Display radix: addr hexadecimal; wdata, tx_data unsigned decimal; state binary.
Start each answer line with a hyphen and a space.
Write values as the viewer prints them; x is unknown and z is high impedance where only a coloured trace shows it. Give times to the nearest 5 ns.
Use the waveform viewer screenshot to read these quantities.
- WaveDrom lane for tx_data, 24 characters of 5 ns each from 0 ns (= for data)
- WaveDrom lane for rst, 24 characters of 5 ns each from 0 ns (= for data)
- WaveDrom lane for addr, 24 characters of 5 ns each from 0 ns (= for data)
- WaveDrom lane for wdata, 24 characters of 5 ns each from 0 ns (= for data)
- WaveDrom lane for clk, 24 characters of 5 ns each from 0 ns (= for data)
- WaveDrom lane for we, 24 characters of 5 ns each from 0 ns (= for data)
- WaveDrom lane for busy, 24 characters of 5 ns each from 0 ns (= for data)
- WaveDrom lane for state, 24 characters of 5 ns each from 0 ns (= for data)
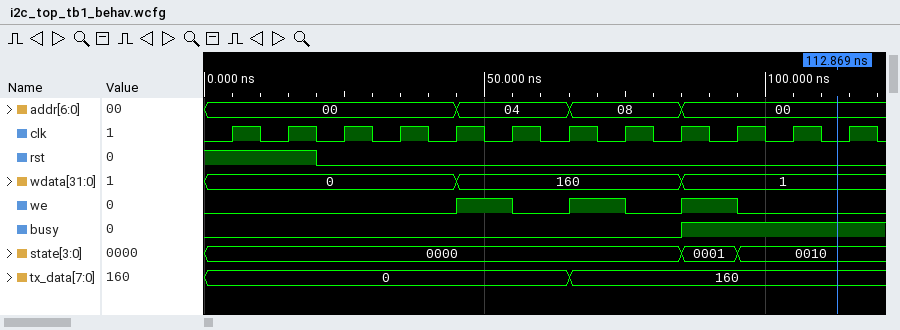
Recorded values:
- {name: 'tx_data', wave: '=............=..........', data: '0 160'}
- {name: 'rst', wave: '1...0...................'}
- {name: 'addr', wave: '=........=...=...=......', data: '00 04 08 00'}
- {name: 'wdata', wave: '=........=.......=......', data: '0 160 1'}
- {name: 'clk', wave: '010101010101010101010101'}
- {name: 'we', wave: '0........1.0.1.0.1.0....'}
- {name: 'busy', wave: '0................1......'}
- {name: 'state', wave: '=................=.=....', data: '0000 0001 0010'}
